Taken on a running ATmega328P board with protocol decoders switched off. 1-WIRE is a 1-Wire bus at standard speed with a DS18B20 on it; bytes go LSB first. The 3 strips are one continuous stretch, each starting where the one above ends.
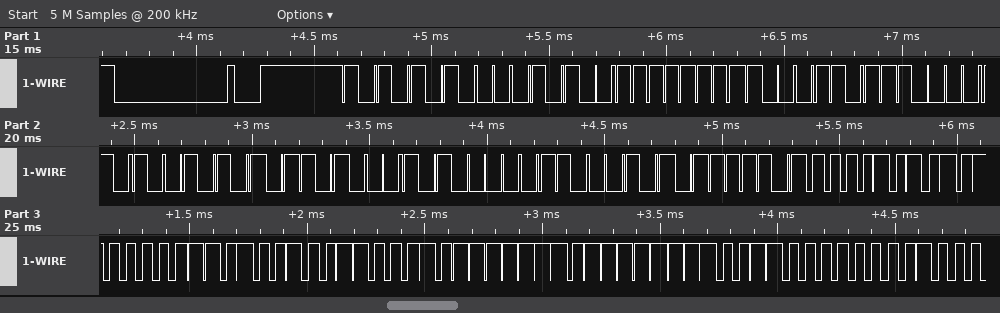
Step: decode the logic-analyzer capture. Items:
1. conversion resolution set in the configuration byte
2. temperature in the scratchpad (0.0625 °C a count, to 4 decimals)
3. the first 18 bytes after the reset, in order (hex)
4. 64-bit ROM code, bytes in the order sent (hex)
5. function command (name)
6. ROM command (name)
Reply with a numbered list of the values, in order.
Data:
1. 12 bits
2. 85.0000 °C
3. 55 28 FF B1 43 A9 16 05 A3 BE 50 05 4B 46 7F FF 0C 10
4. 28 FF B1 43 A9 16 05 A3
5. Read Scratchpad
6. Match ROM
